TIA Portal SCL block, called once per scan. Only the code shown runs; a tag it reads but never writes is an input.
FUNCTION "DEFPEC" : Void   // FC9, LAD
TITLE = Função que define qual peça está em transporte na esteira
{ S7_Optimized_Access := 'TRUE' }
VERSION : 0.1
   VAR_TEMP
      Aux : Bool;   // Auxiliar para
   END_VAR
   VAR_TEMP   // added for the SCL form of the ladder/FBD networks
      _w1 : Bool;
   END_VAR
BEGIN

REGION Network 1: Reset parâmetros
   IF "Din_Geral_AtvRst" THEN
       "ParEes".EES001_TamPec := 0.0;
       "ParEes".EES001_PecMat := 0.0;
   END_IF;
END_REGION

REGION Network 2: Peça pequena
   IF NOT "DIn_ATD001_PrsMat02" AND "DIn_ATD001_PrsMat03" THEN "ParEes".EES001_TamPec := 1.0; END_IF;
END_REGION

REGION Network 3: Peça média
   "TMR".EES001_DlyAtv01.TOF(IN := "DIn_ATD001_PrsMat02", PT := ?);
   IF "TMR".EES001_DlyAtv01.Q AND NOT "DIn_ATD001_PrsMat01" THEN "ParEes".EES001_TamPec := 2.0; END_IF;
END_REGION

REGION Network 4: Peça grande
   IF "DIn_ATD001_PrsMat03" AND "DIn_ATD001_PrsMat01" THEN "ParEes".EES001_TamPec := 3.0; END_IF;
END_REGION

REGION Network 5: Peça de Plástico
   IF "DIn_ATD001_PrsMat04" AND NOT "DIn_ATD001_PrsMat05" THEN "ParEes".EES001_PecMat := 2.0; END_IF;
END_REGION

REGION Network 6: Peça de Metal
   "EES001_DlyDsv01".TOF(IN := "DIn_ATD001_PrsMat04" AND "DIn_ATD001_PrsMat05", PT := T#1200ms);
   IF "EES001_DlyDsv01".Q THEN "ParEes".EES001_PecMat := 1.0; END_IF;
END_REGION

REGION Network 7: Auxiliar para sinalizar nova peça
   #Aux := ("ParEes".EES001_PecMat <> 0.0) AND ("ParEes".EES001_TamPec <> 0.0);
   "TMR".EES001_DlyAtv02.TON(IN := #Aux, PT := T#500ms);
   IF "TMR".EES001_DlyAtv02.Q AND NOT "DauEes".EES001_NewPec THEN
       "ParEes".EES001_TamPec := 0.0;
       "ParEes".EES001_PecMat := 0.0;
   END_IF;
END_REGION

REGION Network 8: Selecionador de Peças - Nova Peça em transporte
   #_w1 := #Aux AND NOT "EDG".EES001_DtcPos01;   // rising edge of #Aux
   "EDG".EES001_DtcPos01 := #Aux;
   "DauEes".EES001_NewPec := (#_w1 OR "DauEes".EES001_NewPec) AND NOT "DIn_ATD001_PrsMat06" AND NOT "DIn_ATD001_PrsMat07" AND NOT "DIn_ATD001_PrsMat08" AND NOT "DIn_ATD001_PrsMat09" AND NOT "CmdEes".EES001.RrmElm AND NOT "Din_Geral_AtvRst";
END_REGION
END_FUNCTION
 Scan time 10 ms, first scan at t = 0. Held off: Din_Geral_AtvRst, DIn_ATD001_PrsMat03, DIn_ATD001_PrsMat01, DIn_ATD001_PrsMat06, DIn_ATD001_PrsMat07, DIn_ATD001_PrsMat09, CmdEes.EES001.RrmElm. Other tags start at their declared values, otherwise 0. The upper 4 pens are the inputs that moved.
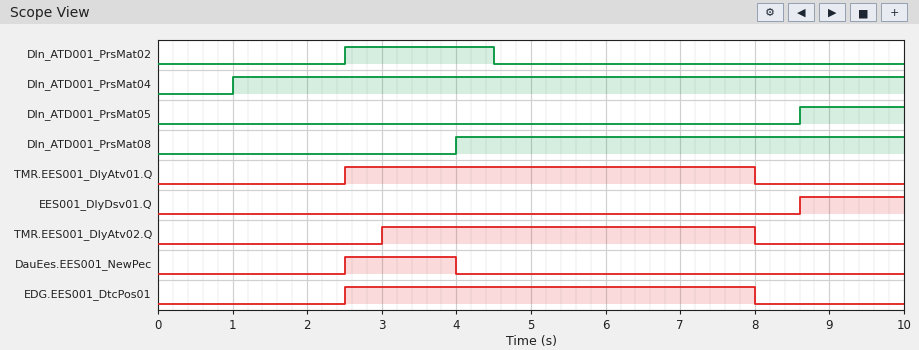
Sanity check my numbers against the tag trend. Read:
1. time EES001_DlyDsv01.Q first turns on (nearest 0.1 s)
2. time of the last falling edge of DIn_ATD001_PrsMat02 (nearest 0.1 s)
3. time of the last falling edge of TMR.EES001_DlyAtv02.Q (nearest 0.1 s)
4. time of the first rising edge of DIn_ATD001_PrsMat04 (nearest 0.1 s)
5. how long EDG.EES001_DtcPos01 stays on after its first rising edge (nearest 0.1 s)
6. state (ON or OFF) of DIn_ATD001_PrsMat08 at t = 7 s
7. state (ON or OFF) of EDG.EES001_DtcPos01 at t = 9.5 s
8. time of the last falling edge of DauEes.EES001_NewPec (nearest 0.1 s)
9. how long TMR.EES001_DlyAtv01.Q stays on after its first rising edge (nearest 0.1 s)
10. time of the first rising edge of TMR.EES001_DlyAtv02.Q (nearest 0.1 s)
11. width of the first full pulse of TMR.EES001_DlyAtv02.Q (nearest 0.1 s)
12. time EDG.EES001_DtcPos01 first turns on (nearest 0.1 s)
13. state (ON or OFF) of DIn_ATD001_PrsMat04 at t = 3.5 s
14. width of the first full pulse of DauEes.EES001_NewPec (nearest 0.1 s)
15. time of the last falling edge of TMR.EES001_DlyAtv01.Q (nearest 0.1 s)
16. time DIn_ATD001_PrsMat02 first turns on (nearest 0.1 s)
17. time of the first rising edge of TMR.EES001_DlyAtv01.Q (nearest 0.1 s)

8.6 s
4.5 s
8.0 s
1.0 s
5.5 s
ON
OFF
4.0 s
5.5 s
3.0 s
5.0 s
2.5 s
ON
1.5 s
8.0 s
2.5 s
2.5 s
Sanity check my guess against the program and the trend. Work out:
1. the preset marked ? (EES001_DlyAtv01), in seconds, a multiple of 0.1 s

3.5 s
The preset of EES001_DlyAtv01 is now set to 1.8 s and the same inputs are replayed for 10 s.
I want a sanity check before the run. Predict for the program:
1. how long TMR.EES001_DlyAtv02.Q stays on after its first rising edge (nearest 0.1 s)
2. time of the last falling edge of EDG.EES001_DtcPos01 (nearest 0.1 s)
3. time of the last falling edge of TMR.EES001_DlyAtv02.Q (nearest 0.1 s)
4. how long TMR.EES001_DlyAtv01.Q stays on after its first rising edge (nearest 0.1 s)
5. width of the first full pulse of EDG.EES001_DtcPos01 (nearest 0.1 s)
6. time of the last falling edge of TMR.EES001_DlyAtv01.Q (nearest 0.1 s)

3.3 s
6.3 s
6.3 s
3.8 s
3.8 s
6.3 s
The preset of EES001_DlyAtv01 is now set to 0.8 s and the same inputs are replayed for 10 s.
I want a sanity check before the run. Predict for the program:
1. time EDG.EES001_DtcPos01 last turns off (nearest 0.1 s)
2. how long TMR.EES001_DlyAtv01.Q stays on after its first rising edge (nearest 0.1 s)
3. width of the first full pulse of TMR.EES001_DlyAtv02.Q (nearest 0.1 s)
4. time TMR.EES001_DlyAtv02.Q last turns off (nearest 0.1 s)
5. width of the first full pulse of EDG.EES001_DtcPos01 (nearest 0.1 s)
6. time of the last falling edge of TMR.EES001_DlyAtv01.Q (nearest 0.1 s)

5.3 s
2.8 s
2.3 s
5.3 s
2.8 s
5.3 s
